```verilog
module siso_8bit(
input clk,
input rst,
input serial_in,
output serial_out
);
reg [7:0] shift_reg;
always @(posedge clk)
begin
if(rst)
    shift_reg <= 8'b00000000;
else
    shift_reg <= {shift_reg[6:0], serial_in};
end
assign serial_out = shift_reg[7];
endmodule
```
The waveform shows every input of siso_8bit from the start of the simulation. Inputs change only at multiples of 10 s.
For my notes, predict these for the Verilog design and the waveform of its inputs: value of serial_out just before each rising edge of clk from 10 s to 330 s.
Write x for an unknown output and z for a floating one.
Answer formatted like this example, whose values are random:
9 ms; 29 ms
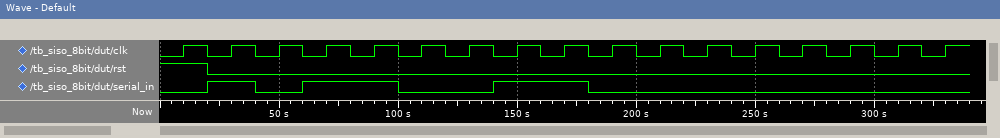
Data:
x 0 0 0 0 0 0 0 0 1 0 1 1 0 0 1 1
